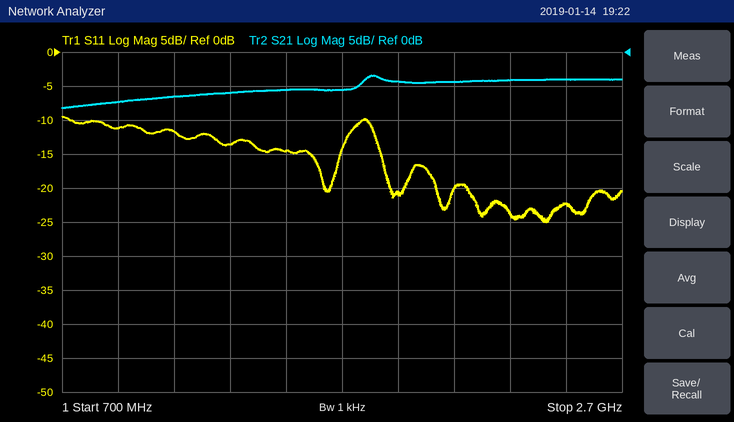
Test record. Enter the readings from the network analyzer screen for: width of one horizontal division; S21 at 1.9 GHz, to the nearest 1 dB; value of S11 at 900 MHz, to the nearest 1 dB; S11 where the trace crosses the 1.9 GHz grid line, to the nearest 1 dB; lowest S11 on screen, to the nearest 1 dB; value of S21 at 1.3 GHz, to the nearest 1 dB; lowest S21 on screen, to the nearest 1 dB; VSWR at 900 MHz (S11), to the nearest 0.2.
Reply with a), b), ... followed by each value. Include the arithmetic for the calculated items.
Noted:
a) 200 MHz
b) -4 dB
c) -11 dB
d) -21 dB
e) -25 dB
f) -6 dB
g) -8 dB
h) |Γ| = 10^(-11/20) = 0.2818; VSWR = (1 + 0.2818)/(1 − 0.2818) ≈ 1.8
